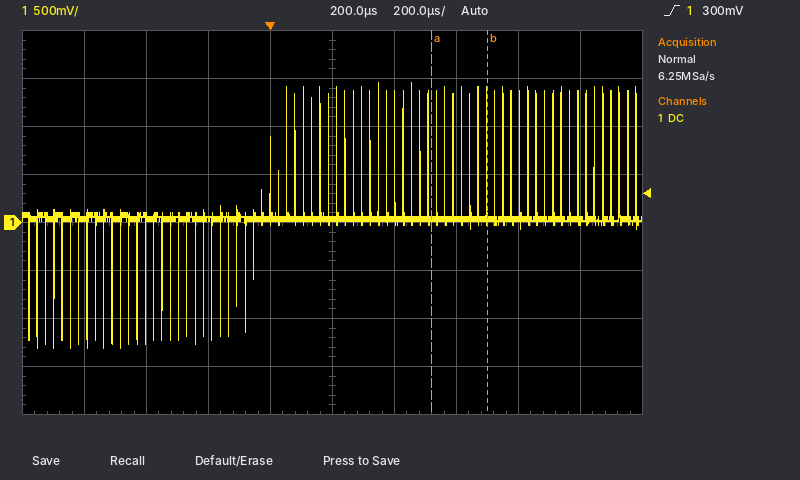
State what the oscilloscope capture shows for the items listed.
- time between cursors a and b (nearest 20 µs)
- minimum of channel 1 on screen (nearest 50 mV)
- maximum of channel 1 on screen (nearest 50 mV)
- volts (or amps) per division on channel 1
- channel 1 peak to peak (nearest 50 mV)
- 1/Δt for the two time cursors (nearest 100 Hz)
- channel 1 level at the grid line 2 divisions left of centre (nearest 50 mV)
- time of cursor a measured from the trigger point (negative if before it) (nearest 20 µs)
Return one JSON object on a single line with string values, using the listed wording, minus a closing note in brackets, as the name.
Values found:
{"time between cursors a and b": "180 µs", "minimum of channel 1 on screen": "-1.30 V", "maximum of channel 1 on screen": "1.45 V", "volts (or amps) per division on channel 1": "500 mV", "channel 1 peak to peak": "2.75 V", "1/Δt for the two time cursors": "5.6 kHz", "channel 1 level at the grid line 2 divisions left of centre": "50 mV", "time of cursor a measured from the trigger point (negative if before it)": "+520 µs"}
